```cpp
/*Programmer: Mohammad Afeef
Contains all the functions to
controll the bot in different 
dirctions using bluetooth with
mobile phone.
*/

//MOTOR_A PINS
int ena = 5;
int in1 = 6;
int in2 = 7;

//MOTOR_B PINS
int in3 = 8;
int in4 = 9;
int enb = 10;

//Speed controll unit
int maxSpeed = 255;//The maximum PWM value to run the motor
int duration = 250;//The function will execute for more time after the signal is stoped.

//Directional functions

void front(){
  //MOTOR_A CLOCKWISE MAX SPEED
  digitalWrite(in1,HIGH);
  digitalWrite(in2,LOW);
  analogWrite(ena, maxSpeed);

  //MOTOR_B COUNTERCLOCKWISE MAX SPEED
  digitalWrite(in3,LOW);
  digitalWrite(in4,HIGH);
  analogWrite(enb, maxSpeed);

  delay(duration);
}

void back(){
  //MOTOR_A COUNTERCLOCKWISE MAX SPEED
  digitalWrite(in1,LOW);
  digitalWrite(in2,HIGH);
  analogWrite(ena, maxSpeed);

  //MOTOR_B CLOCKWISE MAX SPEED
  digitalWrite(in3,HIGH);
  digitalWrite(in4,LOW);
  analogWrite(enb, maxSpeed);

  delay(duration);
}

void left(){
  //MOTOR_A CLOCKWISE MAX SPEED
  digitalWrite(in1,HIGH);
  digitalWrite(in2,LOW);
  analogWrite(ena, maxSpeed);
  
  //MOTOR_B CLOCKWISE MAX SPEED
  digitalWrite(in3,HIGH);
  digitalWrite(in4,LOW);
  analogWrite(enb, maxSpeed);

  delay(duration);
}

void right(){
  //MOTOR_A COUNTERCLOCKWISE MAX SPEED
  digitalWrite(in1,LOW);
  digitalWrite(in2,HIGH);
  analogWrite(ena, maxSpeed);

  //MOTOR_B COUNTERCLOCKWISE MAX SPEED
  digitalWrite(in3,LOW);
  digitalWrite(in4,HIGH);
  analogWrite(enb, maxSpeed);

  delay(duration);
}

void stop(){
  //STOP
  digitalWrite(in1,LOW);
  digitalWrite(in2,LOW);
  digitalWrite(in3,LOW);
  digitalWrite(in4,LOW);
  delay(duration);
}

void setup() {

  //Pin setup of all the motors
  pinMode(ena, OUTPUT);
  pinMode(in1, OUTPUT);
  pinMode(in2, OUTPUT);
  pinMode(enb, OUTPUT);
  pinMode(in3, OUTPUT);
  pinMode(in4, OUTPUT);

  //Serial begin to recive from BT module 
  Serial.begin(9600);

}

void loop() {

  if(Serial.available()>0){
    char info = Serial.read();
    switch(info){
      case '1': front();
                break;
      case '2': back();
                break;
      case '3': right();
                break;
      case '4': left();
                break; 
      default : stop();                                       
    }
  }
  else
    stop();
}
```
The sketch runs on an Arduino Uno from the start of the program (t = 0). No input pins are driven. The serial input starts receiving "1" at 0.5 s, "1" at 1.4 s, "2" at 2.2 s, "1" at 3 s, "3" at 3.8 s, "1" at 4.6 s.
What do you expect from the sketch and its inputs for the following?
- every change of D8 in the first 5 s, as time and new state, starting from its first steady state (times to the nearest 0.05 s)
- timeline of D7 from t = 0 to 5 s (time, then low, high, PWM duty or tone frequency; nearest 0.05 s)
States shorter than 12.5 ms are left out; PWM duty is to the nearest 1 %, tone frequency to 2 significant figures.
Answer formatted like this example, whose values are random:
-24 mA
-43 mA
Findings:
0 s low; 2.25 s high; 2.5 s low
0 s low; 2.25 s high; 2.5 s low; 4 s high; 4.25 s low
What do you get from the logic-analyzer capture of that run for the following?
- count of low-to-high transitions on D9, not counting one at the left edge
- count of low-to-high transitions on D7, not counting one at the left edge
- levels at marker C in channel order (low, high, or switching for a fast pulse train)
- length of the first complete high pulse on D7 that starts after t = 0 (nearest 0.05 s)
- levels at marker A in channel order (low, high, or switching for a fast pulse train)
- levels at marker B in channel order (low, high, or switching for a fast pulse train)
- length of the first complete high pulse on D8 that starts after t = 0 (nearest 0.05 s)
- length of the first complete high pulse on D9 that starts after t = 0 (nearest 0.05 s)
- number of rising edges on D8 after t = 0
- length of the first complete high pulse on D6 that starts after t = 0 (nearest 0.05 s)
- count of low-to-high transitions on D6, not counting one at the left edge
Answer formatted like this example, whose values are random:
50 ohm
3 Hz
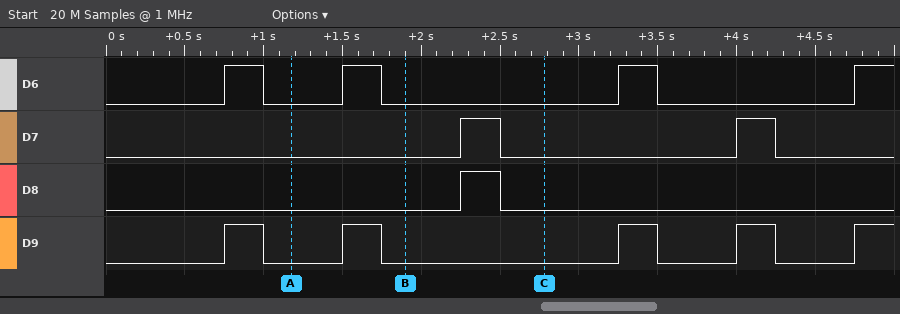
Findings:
5
2
D6 low, D7 low, D8 low, D9 low
0.25 s
D6 low, D7 low, D8 low, D9 low
D6 low, D7 low, D8 low, D9 low
0.25 s
0.25 s
1
0.25 s
4
